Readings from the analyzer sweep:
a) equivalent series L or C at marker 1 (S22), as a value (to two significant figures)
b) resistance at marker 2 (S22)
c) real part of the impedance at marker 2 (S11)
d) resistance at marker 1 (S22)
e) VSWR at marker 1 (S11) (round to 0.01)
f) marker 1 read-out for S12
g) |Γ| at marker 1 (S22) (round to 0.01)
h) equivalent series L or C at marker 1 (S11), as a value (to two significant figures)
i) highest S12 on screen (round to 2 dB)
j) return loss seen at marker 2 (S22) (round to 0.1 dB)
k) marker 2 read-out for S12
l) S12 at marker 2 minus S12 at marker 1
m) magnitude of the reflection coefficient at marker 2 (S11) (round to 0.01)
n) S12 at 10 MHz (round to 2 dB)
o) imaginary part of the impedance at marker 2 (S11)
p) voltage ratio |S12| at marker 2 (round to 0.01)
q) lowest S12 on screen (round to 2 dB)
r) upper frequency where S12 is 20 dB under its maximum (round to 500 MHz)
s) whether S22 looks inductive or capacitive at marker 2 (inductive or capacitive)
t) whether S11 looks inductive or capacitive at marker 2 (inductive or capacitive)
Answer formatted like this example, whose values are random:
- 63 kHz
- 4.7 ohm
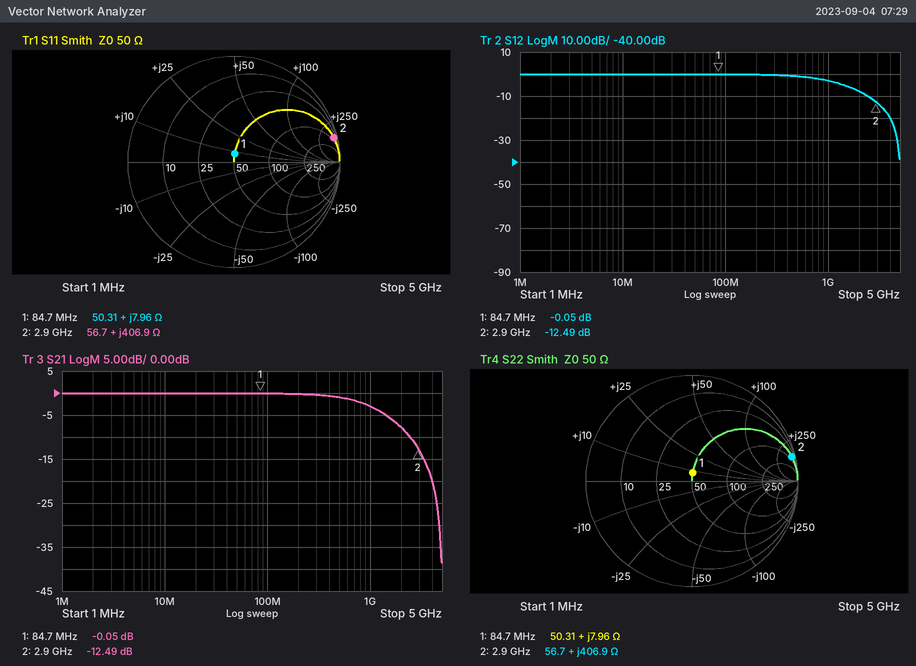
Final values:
- 15 nH
- 56.7 Ω
- 56.7 Ω
- 50.31 Ω
- 1.17
- -0.05 dB
- 0.08
- 15 nH
- 0 dB
- 0.3 dB
- -12.49 dB
- -12.44 dB
- 0.97
- 0 dB
- +406.9 Ω
- 0.24
- -38 dB
- 4.0 GHz
- inductive
- inductive
